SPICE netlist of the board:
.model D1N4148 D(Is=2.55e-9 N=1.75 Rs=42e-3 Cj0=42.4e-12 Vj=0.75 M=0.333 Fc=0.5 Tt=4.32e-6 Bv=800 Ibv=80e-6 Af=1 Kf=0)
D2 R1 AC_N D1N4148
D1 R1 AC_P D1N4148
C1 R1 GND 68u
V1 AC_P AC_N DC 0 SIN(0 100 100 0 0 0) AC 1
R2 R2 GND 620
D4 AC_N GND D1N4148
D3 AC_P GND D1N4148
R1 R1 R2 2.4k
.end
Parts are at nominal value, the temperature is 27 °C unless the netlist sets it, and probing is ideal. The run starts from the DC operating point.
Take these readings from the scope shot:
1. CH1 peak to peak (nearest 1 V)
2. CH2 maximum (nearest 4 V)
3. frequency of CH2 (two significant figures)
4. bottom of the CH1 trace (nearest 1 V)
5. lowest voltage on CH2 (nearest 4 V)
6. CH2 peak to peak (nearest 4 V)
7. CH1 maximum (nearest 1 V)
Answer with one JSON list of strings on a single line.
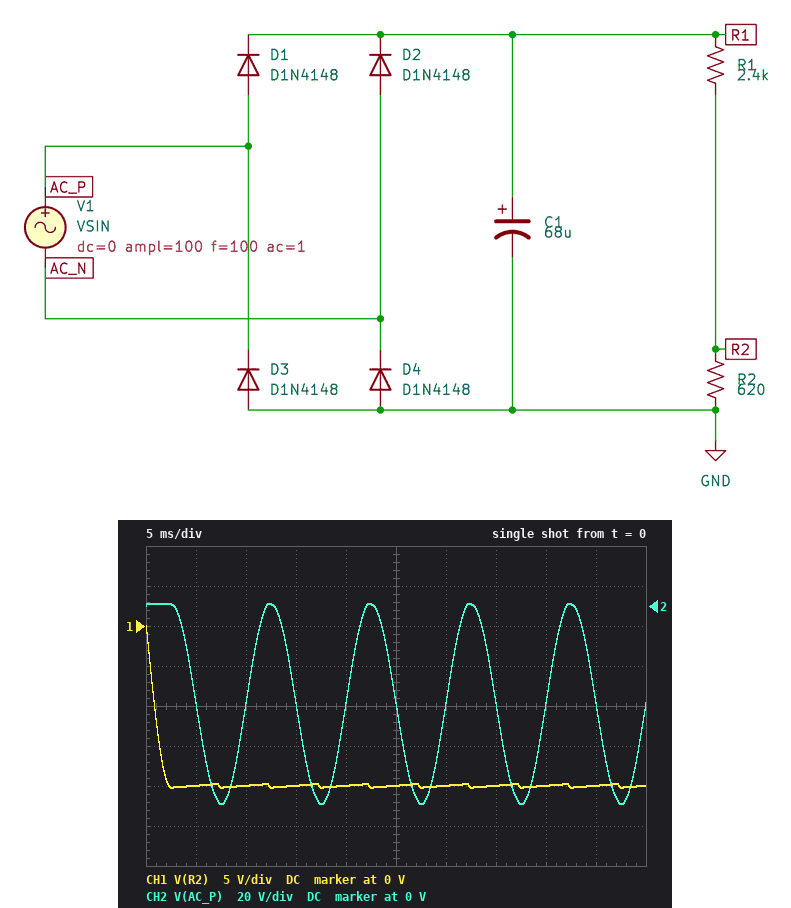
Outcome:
["20 V", "0 V", "100 Hz", "-20 V", "-100 V", "100 V", "0 V"]
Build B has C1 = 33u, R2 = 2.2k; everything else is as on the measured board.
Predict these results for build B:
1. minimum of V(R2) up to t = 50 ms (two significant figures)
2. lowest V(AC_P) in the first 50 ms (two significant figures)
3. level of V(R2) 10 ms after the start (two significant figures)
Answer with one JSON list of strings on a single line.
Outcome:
["-47 V", "-99 V", "-46 V"]
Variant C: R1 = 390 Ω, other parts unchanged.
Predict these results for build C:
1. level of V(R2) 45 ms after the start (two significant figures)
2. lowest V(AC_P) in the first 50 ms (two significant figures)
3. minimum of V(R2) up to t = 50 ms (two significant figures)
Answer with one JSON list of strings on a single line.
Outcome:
["-58 V", "-99 V", "-60 V"]
